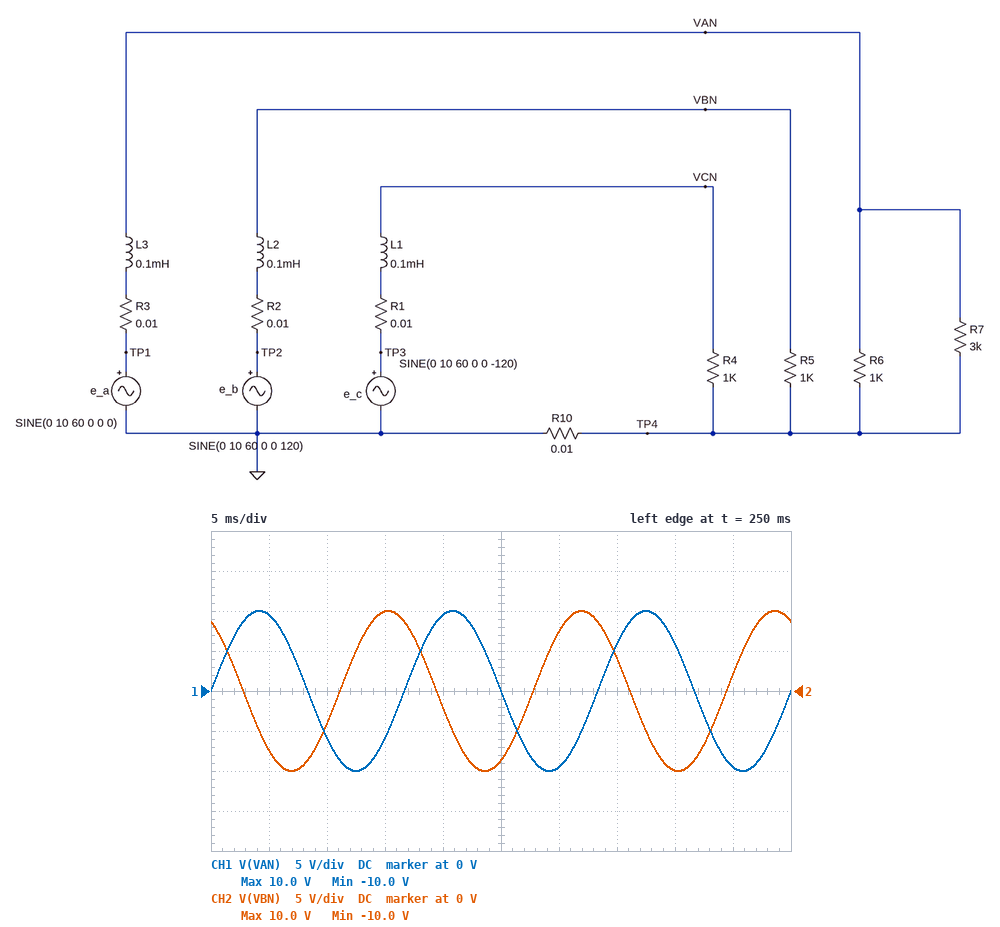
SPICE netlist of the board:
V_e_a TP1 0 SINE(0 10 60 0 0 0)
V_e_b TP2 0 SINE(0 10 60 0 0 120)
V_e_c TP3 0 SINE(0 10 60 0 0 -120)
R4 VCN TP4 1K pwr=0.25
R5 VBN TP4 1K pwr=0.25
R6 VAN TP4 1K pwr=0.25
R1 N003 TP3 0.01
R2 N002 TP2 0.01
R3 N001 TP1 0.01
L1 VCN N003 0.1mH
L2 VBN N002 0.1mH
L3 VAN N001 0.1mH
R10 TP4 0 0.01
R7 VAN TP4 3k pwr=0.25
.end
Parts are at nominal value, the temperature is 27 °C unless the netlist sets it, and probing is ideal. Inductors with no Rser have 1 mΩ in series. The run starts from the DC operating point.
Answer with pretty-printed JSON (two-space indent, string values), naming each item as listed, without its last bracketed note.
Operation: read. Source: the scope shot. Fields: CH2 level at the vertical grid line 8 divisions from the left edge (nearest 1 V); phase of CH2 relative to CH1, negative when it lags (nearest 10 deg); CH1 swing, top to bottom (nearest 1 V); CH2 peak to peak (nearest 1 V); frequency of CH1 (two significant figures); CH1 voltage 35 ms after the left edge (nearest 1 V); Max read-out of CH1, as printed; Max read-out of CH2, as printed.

{
  "CH2 level at the vertical grid line 8 divisions from the left edge": "-10 V",
  "phase of CH2 relative to CH1, negative when it lags": "120 deg",
  "CH1 swing, top to bottom": "20 V",
  "CH2 peak to peak": "20 V",
  "frequency of CH1": "60 Hz",
  "CH1 voltage 35 ms after the left edge": "6 V",
  "Max read-out of CH1, as printed": "10.0 V",
  "Max read-out of CH2, as printed": "10.0 V"
}
